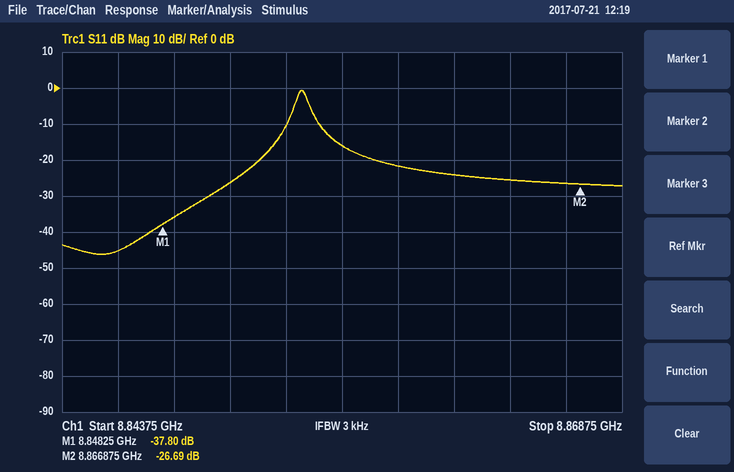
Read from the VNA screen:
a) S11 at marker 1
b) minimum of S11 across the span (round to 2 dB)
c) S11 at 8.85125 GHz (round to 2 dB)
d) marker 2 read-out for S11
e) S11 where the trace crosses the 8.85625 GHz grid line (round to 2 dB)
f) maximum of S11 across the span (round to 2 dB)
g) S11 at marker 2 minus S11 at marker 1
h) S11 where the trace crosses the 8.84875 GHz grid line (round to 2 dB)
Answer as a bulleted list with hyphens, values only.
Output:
- -37.80 dB
- -46 dB
- -26 dB
- -26.69 dB
- -16 dB
- 0 dB
- 11.11 dB
- -36 dB
